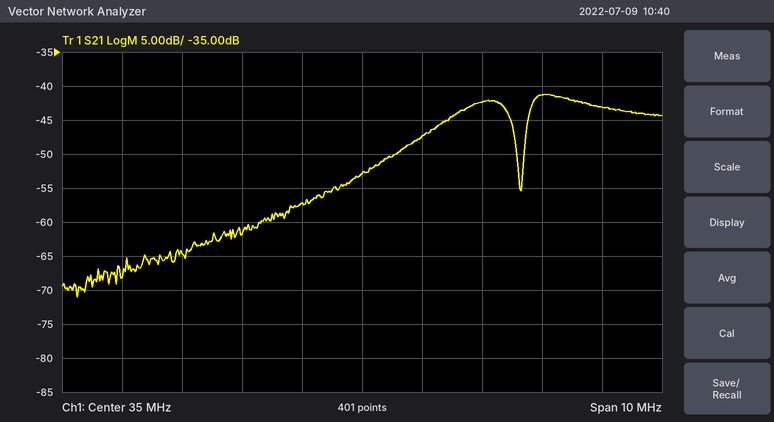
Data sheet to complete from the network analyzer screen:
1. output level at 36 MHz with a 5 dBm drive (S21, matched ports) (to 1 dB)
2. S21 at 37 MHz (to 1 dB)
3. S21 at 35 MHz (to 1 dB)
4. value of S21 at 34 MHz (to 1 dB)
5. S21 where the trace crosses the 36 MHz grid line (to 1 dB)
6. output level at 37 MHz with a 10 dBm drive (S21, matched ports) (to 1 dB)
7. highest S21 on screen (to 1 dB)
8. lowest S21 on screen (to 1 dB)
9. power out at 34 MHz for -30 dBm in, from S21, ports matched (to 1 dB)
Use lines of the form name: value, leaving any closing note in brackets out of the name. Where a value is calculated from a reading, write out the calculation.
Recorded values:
output level at 36 MHz with a 5 dBm drive (S21, matched ports): 5 dBm + (-47 dB) = -42 dBm
S21 at 37 MHz: -42 dB
S21 at 35 MHz: -53 dB
value of S21 at 34 MHz: -57 dB
S21 where the trace crosses the 36 MHz grid line: -47 dB
output level at 37 MHz with a 10 dBm drive (S21, matched ports): 10 dBm + (-42 dB) = -32 dBm
highest S21 on screen: -41 dB
lowest S21 on screen: -71 dB
power out at 34 MHz for -30 dBm in, from S21, ports matched: -30 dBm + (-57 dB) = -87 dBm
